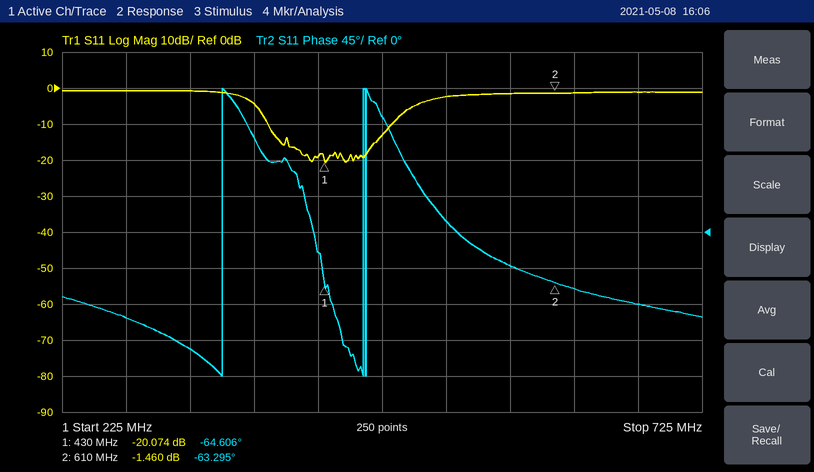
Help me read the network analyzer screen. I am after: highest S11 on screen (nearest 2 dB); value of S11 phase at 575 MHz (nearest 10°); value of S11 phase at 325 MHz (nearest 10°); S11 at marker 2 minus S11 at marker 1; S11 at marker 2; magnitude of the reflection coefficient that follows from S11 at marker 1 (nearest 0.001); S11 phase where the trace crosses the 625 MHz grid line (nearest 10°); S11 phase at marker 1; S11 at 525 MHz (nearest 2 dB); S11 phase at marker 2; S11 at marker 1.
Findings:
0 dB
-40°
-150°
18.614 dB
-1.460 dB
0.099
-70°
-64.606°
-2 dB
-63.295°
-20.074 dB
